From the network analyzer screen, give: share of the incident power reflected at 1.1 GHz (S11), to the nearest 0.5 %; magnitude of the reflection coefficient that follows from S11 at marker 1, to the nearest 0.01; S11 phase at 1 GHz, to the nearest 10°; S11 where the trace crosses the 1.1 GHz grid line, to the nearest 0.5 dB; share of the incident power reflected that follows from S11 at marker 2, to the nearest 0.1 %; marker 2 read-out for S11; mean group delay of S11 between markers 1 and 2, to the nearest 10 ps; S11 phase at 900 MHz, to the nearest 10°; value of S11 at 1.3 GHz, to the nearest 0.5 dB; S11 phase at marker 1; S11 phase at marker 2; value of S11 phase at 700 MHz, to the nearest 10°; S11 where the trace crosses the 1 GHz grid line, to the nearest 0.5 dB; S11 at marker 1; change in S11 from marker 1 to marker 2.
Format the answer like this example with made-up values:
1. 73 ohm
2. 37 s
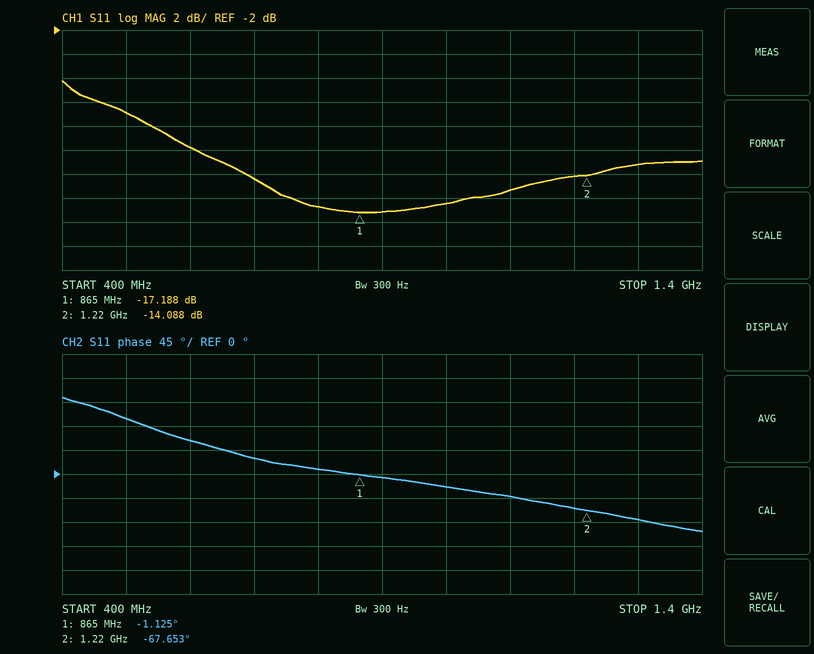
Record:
1. 3.0 %
2. 0.14
3. -20°
4. -15.5 dB
5. 3.9 %
6. -14.088 dB
7. 520 ps
8. -10°
9. -13.0 dB
10. -1.125°
11. -67.653°
12. 30°
13. -16.5 dB
14. -17.188 dB
15. 3.100 dB
